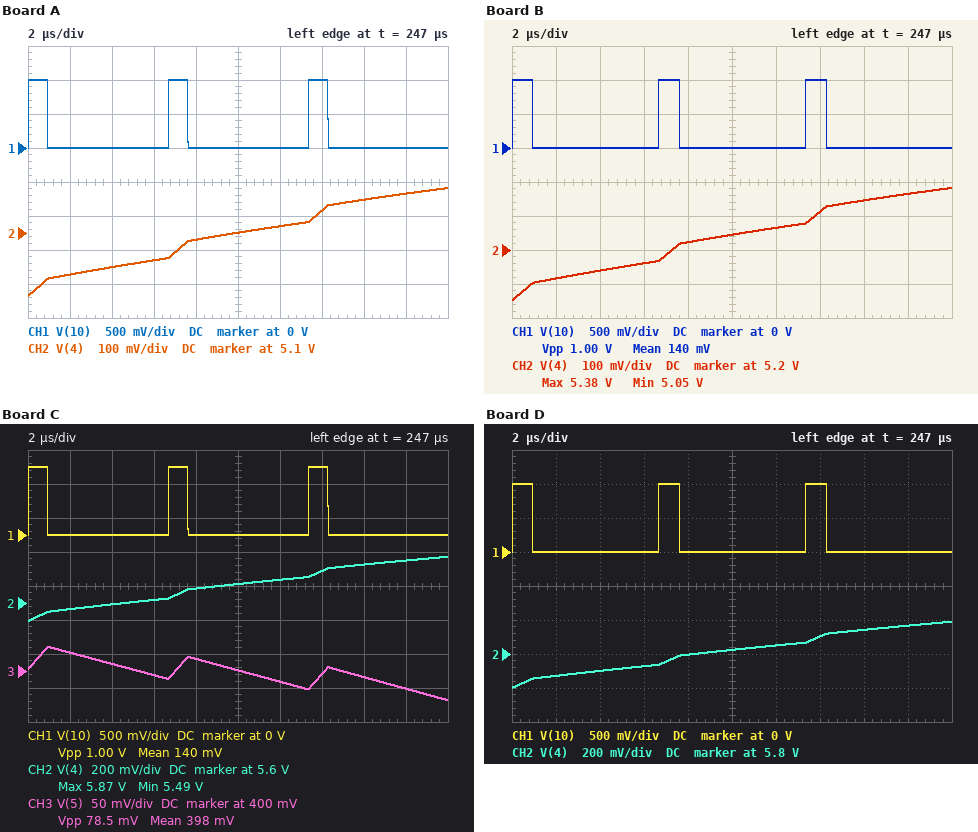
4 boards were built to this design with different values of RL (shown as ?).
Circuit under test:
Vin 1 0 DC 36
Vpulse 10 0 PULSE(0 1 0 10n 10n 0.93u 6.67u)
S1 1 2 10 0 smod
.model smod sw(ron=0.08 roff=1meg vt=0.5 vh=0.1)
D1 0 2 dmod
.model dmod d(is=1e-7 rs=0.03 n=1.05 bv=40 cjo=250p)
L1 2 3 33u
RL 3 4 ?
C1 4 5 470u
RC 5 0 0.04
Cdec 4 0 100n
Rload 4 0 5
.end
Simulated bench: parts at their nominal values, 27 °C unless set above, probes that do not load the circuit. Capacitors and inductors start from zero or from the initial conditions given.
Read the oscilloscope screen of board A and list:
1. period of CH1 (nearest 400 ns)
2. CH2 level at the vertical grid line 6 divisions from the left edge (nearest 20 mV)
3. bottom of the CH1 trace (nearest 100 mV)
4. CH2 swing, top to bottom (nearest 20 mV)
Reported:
6.8 µs
5.12 V
0 V
320 mV
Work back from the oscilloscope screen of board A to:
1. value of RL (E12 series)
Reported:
0.082 Ω
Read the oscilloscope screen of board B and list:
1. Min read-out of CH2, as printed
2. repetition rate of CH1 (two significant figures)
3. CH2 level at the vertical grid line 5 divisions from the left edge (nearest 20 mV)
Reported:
5.05 V
150 kHz
5.24 V
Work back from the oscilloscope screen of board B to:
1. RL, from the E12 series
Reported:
0.068 Ω
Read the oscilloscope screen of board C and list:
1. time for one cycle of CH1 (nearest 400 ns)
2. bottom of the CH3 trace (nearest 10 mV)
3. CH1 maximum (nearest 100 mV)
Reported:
6.8 µs
360 mV
1.0 V
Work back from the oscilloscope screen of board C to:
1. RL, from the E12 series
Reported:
0.027 Ω
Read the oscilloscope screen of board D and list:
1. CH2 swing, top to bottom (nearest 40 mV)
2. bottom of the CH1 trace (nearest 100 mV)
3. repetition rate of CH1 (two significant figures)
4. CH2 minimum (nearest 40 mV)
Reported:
400 mV
0 V
150 kHz
5.60 V
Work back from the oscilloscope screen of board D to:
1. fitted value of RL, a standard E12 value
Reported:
0.018 Ω
